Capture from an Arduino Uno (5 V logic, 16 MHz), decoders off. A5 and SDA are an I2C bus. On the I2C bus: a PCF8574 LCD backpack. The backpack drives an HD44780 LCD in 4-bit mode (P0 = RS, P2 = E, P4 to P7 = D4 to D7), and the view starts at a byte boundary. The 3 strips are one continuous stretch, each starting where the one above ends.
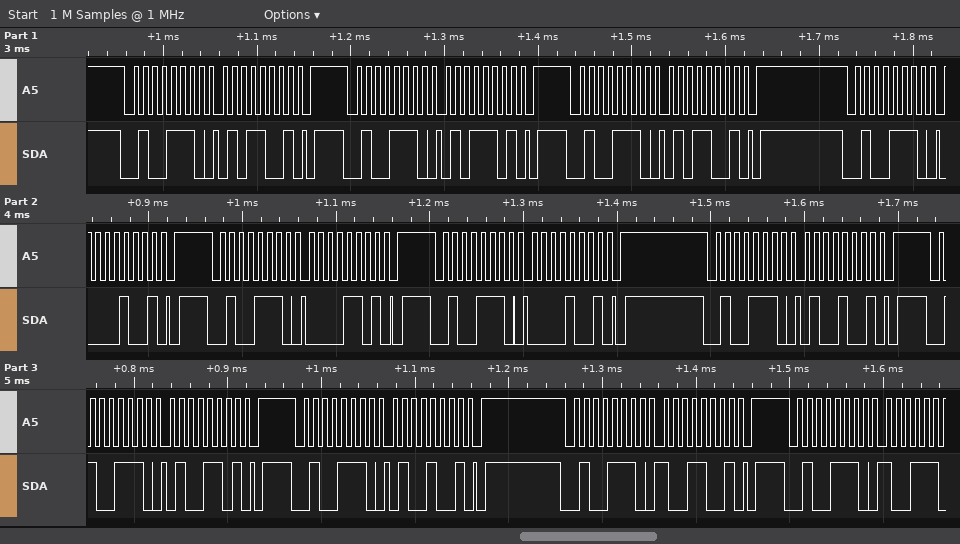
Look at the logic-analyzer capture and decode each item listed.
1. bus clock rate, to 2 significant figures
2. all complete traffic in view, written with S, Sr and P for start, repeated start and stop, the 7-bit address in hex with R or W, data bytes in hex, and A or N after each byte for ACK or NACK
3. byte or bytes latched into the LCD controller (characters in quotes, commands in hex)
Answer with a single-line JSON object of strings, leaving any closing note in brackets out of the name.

{"bus clock rate, to 2 significant figures": "100 kHz", "all complete traffic in view, written with S, Sr and P for start, repeated start and stop, the 7-bit address in hex with R or W, data bytes in hex, and A or N after each byte for ACK or NACK": "S 27W A 59 A P S 27W A 5D A P S 27W A 59 A P S 27W A 09 A P S 27W A 0D A P S 27W A 09 A P S 27W A 49 A P S 27W A 4D A P S 27W A 49 A P S 27W A 99 A P S 27W A", "byte or bytes latched into the LCD controller": "'P'"}
